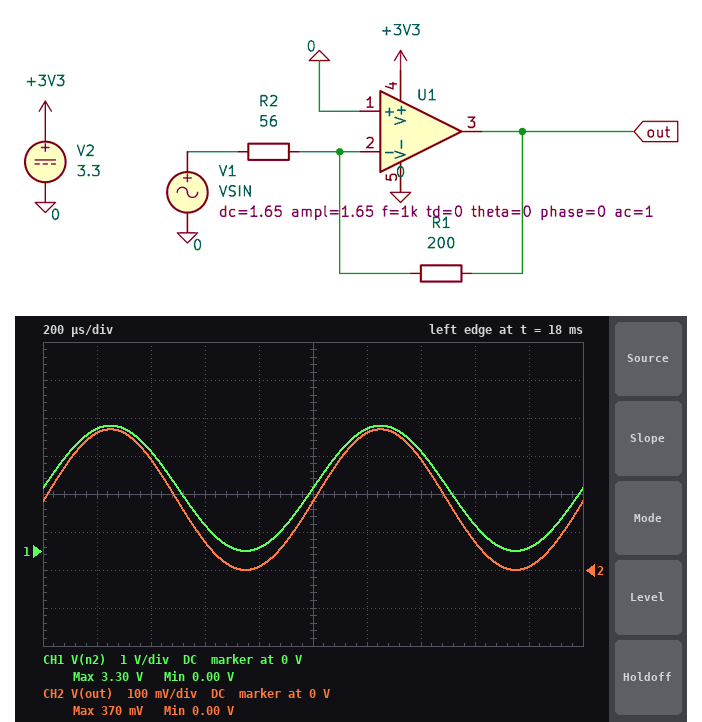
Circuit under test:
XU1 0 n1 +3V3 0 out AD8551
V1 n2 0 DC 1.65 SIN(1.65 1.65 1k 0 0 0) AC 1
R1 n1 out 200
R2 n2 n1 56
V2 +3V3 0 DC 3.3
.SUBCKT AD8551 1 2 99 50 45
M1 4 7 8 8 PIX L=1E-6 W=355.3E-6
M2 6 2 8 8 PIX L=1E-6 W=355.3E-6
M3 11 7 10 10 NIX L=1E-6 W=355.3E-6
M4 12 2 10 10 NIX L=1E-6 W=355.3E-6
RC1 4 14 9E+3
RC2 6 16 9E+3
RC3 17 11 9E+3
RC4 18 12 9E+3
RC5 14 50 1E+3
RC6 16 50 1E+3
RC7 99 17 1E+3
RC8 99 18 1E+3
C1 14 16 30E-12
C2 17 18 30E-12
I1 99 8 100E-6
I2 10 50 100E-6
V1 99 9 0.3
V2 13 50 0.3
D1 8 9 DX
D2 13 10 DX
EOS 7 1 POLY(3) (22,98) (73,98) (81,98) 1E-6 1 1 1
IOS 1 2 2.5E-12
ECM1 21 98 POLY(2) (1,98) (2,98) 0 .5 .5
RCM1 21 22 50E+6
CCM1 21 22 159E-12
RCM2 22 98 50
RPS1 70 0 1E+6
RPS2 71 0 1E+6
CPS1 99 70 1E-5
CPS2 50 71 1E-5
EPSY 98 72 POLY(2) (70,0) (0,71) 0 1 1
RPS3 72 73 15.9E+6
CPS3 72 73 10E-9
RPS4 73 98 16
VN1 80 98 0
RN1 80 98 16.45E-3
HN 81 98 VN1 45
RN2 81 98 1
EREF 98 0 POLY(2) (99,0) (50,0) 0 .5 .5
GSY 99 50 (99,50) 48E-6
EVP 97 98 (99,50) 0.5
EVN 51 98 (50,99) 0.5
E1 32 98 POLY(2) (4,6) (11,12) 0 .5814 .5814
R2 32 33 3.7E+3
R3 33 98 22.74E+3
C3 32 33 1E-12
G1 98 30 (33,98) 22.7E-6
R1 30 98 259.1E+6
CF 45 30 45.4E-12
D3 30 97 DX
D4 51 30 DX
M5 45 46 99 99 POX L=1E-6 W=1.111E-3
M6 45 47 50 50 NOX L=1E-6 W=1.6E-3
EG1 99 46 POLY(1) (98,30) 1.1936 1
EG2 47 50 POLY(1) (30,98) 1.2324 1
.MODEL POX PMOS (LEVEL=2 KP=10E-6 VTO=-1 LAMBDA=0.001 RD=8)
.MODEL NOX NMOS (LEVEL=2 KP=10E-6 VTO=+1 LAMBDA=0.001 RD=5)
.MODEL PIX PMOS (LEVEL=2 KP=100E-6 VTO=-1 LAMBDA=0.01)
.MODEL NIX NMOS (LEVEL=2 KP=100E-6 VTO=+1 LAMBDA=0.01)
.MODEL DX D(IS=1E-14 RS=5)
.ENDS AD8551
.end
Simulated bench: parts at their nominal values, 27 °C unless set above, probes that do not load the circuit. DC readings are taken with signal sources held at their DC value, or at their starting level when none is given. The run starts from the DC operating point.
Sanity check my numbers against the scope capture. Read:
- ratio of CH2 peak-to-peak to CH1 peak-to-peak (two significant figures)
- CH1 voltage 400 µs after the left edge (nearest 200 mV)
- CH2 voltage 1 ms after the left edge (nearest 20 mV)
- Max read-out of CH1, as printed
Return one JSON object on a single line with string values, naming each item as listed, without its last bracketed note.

{"ratio of CH2 peak-to-peak to CH1 peak-to-peak": "0.11", "CH1 voltage 400 µs after the left edge": "2.6 V", "CH2 voltage 1 ms after the left edge": "180 mV", "Max read-out of CH1, as printed": "3.30 V"}
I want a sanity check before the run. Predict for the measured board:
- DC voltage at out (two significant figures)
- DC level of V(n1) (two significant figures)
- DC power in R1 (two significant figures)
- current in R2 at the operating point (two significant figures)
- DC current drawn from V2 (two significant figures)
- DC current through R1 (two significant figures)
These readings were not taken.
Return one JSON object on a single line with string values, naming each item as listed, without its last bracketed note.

{"DC voltage at out": "180 mV", "DC level of V(n1)": "1.3 V", "DC power in R1": "6.6 mW", "current in R2 at the operating point": "5.7 mA", "DC current drawn from V2": "360 µA", "DC current through R1": "5.7 mA"}
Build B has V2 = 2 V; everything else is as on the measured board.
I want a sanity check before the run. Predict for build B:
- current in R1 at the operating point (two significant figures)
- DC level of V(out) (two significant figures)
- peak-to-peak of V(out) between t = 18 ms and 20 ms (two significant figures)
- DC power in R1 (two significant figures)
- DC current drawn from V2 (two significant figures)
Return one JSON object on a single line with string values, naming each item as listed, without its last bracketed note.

{"current in R1 at the operating point": "5.5 mA", "DC level of V(out)": "230 mV", "peak-to-peak of V(out) between t = 18 ms and 20 ms": "490 mV", "DC power in R1": "6.1 mW", "DC current drawn from V2": "300 µA"}
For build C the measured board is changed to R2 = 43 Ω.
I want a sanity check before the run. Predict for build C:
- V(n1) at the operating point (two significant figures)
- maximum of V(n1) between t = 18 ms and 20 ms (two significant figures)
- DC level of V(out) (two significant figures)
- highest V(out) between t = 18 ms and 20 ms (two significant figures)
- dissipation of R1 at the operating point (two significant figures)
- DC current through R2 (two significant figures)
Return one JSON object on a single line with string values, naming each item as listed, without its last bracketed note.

{"V(n1) at the operating point": "1.4 V", "maximum of V(n1) between t = 18 ms and 20 ms": "2.8 V", "DC level of V(out)": "190 mV", "highest V(out) between t = 18 ms and 20 ms": "390 mV", "dissipation of R1 at the operating point": "7.2 mW", "DC current through R2": "6.0 mA"}
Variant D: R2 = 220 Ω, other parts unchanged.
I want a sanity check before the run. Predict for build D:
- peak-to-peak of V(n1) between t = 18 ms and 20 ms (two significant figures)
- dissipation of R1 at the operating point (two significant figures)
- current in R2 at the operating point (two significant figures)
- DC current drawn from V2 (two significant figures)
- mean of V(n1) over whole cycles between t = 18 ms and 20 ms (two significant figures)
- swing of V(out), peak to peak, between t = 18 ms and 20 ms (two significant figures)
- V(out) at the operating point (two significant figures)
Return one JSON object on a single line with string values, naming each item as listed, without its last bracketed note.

{"peak-to-peak of V(n1) between t = 18 ms and 20 ms": "1.7 V", "dissipation of R1 at the operating point": "2.7 mW", "current in R2 at the operating point": "3.7 mA", "DC current drawn from V2": "350 µA", "mean of V(n1) over whole cycles between t = 18 ms and 20 ms": "850 mV", "swing of V(out), peak to peak, between t = 18 ms and 20 ms": "230 mV", "V(out) at the operating point": "110 mV"}
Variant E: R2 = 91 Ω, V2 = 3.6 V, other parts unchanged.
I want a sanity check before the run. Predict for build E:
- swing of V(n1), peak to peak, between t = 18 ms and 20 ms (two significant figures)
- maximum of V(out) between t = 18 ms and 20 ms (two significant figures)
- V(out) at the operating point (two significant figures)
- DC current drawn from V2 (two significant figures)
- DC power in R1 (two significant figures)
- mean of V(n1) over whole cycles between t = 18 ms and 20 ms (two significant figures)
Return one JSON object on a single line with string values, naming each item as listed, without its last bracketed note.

{"swing of V(n1), peak to peak, between t = 18 ms and 20 ms": "2.4 V", "maximum of V(out) between t = 18 ms and 20 ms": "310 mV", "V(out) at the operating point": "150 mV", "DC current drawn from V2": "370 µA", "DC power in R1": "5.3 mW", "mean of V(n1) over whole cycles between t = 18 ms and 20 ms": "1.2 V"}
